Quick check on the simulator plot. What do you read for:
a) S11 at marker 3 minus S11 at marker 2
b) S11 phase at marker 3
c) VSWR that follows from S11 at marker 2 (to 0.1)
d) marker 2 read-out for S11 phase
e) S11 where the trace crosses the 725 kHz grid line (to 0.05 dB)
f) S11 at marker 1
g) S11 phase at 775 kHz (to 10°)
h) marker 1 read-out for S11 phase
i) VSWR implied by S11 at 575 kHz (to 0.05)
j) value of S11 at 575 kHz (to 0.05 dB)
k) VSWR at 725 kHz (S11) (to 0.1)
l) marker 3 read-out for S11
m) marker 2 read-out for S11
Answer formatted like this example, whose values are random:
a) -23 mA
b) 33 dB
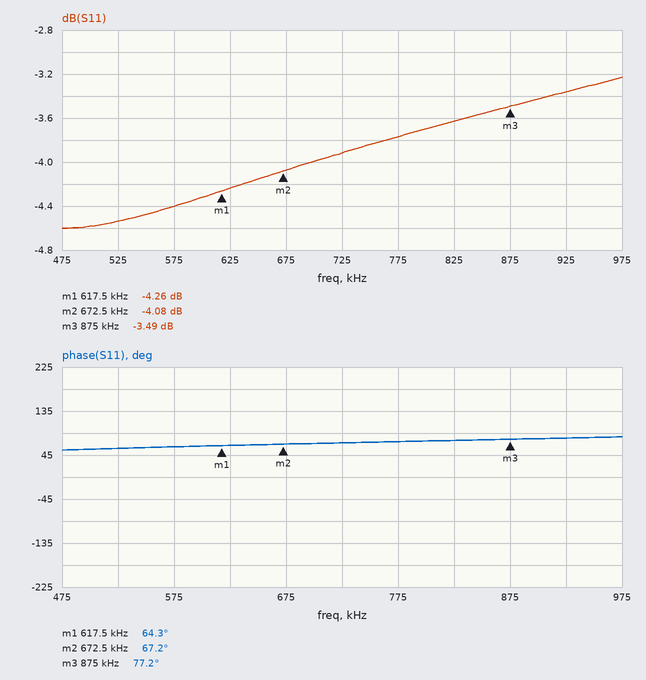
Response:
a) 0.59 dB
b) 77.2°
c) 4.3
d) 67.2°
e) -3.90 dB
f) -4.26 dB
g) 70°
h) 64.3°
i) 4.05
j) -4.40 dB
k) 4.5
l) -3.49 dB
m) -4.08 dB
